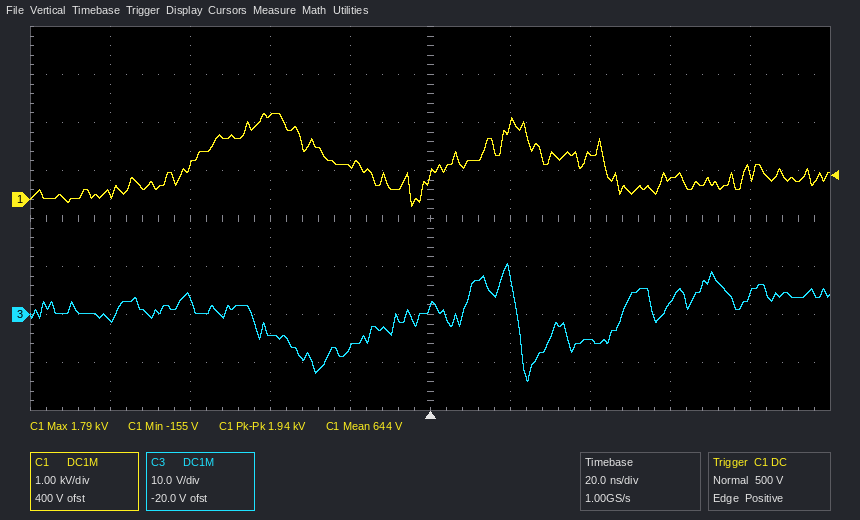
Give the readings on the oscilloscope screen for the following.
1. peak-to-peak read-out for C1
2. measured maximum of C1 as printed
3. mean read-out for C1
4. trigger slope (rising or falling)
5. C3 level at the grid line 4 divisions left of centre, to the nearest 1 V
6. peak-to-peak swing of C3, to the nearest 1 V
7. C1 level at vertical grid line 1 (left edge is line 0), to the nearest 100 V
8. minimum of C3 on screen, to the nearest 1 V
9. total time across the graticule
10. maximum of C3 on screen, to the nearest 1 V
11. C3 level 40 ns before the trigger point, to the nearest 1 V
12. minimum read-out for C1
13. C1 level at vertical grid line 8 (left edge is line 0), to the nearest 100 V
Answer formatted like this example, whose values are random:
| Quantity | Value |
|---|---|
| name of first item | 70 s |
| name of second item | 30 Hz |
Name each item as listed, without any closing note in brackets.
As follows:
| Quantity | Value |
|---|---|
| peak-to-peak read-out for C1 | 1.94 kV |
| measured maximum of C1 as printed | 1.79 kV |
| mean read-out for C1 | 644 V |
| trigger slope | rising |
| C3 level at the grid line 4 divisions left of centre, to the nearest 1 V | -1 V |
| peak-to-peak swing of C3, to the nearest 1 V | 25 V |
| C1 level at vertical grid line 1 (left edge is line 0), to the nearest 100 V | 100 V |
| minimum of C3 on screen, to the nearest 1 V | -14 V |
| total time across the graticule | 200 ns |
| maximum of C3 on screen, to the nearest 1 V | 11 V |
| C3 level 40 ns before the trigger point, to the nearest 1 V | -4 V |
| minimum read-out for C1 | -155 V |
| C1 level at vertical grid line 8 (left edge is line 0), to the nearest 100 V | 400 V |
